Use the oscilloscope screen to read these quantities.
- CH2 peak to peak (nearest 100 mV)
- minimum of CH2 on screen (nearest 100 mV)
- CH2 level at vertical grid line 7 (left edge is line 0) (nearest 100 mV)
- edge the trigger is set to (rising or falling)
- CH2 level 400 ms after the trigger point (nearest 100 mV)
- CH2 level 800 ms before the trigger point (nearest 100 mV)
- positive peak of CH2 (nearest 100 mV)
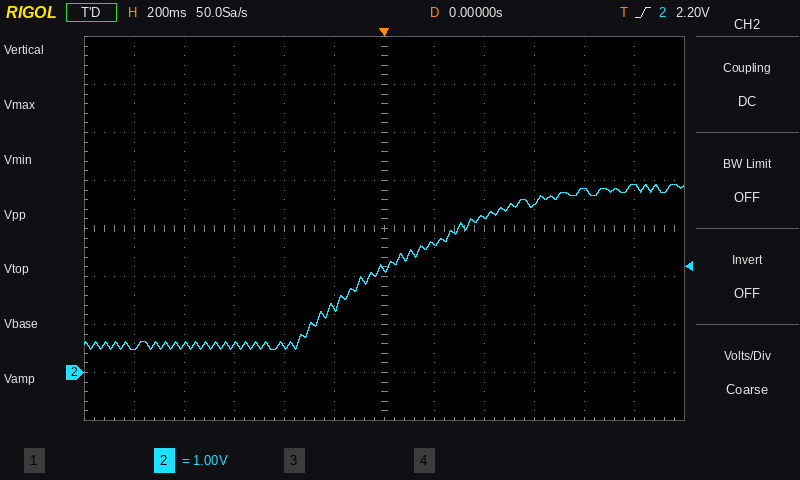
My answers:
3.4 V
500 mV
2.7 V
rising
3.2 V
600 mV
3.9 V
